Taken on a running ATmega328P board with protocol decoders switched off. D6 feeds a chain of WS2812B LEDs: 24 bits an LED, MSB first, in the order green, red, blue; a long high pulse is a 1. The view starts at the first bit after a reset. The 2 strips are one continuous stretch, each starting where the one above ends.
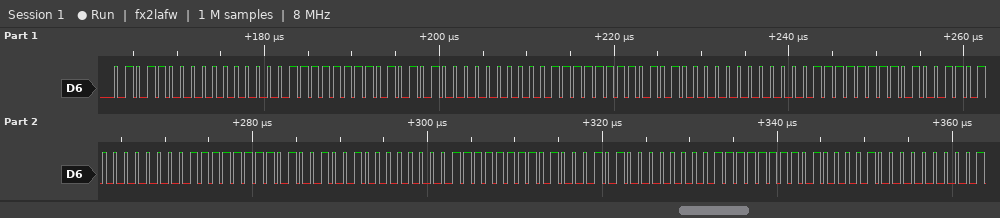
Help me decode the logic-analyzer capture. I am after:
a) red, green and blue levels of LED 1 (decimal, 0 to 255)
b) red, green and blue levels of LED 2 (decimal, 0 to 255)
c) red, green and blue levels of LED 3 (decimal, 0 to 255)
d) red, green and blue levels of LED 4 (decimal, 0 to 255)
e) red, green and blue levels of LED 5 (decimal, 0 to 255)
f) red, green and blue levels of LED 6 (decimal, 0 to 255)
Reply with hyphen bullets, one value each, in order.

- 0, 88, 255
- 0, 84, 255
- 0, 80, 255
- 0, 77, 255
- 0, 73, 255
- 0, 69, 255
